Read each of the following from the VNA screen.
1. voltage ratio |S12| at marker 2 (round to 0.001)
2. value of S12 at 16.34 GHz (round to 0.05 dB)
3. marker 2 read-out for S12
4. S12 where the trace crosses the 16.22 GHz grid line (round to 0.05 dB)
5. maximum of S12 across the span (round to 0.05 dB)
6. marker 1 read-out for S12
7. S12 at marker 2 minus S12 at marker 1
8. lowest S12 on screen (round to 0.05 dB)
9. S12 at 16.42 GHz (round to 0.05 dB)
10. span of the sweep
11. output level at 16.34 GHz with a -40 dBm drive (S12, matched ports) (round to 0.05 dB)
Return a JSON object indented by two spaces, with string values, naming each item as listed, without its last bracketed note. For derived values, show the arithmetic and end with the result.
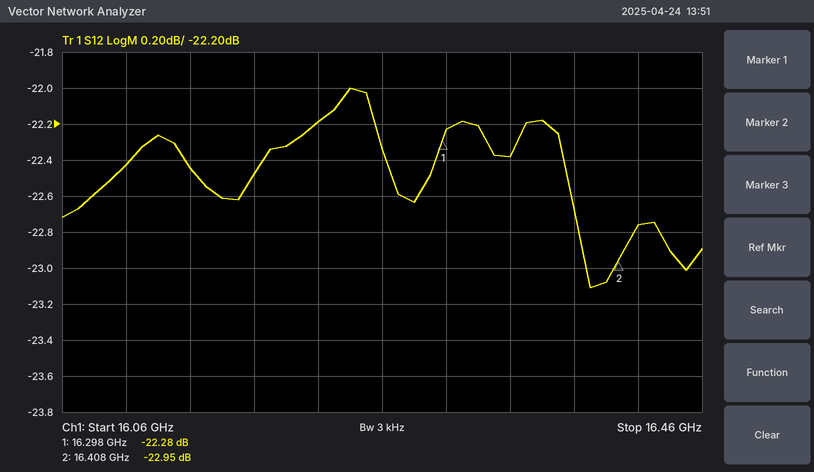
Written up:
{
  "voltage ratio |S12| at marker 2": "10^(-22.95/20) ≈ 0.071",
  "value of S12 at 16.34 GHz": "-22.40 dB",
  "marker 2 read-out for S12": "-22.95 dB",
  "S12 where the trace crosses the 16.22 GHz grid line": "-22.20 dB",
  "maximum of S12 across the span": "-22.00 dB",
  "marker 1 read-out for S12": "-22.28 dB",
  "S12 at marker 2 minus S12 at marker 1": "-22.95 − (-22.28) = -0.67 dB",
  "lowest S12 on screen": "-23.10 dB",
  "S12 at 16.42 GHz": "-22.75 dB",
  "span of the sweep": "400 MHz",
  "output level at 16.34 GHz with a -40 dBm drive (S12, matched ports)": "-40 dBm + (-22.40 dB) = -62.40 dBm"
}
